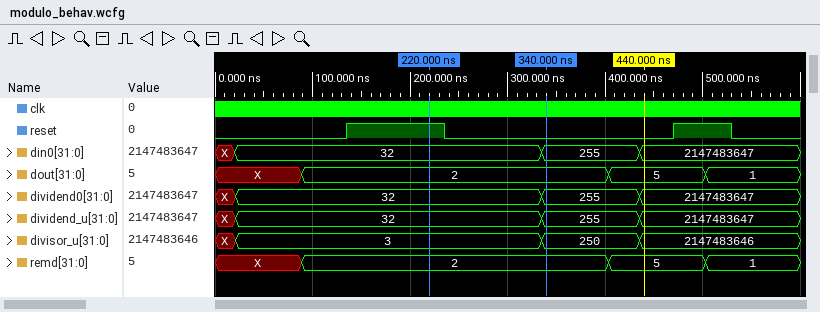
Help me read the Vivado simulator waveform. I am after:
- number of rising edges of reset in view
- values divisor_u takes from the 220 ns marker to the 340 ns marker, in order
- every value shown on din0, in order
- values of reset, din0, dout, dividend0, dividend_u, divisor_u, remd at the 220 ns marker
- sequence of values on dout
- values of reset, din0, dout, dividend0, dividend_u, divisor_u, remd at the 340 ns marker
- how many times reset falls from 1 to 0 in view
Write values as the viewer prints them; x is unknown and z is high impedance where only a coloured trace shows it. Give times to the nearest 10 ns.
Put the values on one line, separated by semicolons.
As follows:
2; 3, 250; X, 32, 255, 2147483647; reset=1, din0=32, dout=2, dividend0=32, dividend_u=32, divisor_u=3, remd=2; X, 2, 5, 1; reset=0, din0=255, dout=2, dividend0=255, dividend_u=255, divisor_u=250, remd=2; 2
